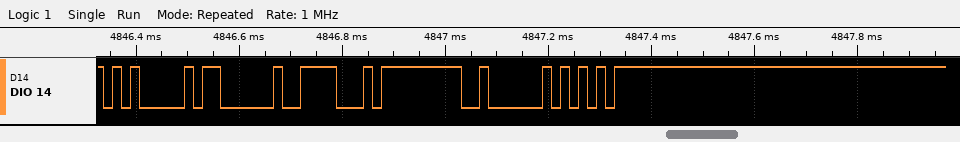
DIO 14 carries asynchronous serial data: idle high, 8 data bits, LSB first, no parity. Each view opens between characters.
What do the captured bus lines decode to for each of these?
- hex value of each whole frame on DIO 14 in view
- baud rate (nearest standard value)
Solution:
05, 03, 1E, FF, 02, D5
57600 baud
